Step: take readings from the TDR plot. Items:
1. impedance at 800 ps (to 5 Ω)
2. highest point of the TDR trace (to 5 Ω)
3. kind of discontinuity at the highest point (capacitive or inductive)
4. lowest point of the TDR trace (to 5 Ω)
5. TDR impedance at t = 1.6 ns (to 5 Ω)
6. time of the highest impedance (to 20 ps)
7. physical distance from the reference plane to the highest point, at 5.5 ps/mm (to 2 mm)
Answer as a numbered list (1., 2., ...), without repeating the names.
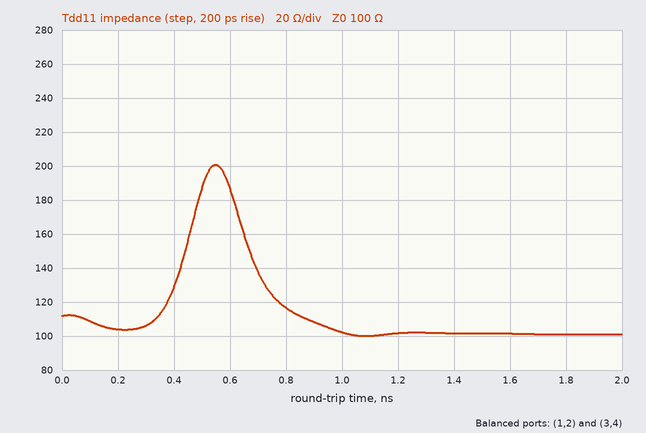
1. 115 Ω
2. 200 Ω
3. inductive
4. 100 Ω
5. 100 Ω
6. 540 ps
7. 50 mm
